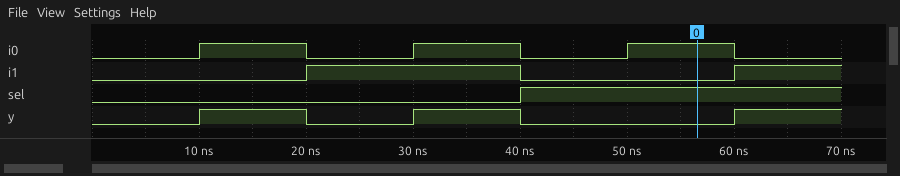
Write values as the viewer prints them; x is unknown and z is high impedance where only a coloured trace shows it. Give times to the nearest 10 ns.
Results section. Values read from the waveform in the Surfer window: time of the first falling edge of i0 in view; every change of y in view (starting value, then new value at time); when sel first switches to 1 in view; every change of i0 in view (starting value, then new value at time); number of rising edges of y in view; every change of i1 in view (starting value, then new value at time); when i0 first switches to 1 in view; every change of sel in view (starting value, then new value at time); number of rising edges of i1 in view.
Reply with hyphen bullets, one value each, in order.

- 20 ns
- 0, 1 at 10 ns, 0 at 20 ns, 1 at 30 ns, 0 at 40 ns, 1 at 60 ns
- 40 ns
- 0, 1 at 10 ns, 0 at 20 ns, 1 at 30 ns, 0 at 40 ns, 1 at 50 ns, 0 at 60 ns
- 3
- 0, 1 at 20 ns, 0 at 40 ns, 1 at 60 ns
- 10 ns
- 0, 1 at 40 ns
- 2
